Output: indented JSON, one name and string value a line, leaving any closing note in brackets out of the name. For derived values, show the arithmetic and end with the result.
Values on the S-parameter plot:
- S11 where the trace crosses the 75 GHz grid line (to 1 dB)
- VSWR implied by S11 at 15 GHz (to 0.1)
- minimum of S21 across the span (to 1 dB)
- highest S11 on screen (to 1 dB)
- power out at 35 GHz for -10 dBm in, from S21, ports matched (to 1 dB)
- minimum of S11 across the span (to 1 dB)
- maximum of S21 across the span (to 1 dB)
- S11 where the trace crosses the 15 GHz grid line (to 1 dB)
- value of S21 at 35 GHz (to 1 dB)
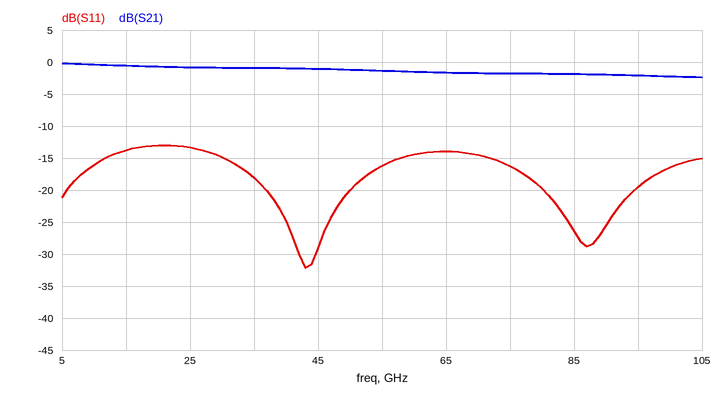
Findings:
{
  "S11 where the trace crosses the 75 GHz grid line": "-16 dB",
  "VSWR implied by S11 at 15 GHz": "|Γ| = 10^(-14/20) = 0.1995; VSWR = (1 + 0.1995)/(1 − 0.1995) ≈ 1.5",
  "minimum of S21 across the span": "-2 dB",
  "highest S11 on screen": "-13 dB",
  "power out at 35 GHz for -10 dBm in, from S21, ports matched": "-10 dBm + (-1 dB) = -11 dBm",
  "minimum of S11 across the span": "-32 dB",
  "maximum of S21 across the span": "0 dB",
  "S11 where the trace crosses the 15 GHz grid line": "-14 dB",
  "value of S21 at 35 GHz": "-1 dB"
}
